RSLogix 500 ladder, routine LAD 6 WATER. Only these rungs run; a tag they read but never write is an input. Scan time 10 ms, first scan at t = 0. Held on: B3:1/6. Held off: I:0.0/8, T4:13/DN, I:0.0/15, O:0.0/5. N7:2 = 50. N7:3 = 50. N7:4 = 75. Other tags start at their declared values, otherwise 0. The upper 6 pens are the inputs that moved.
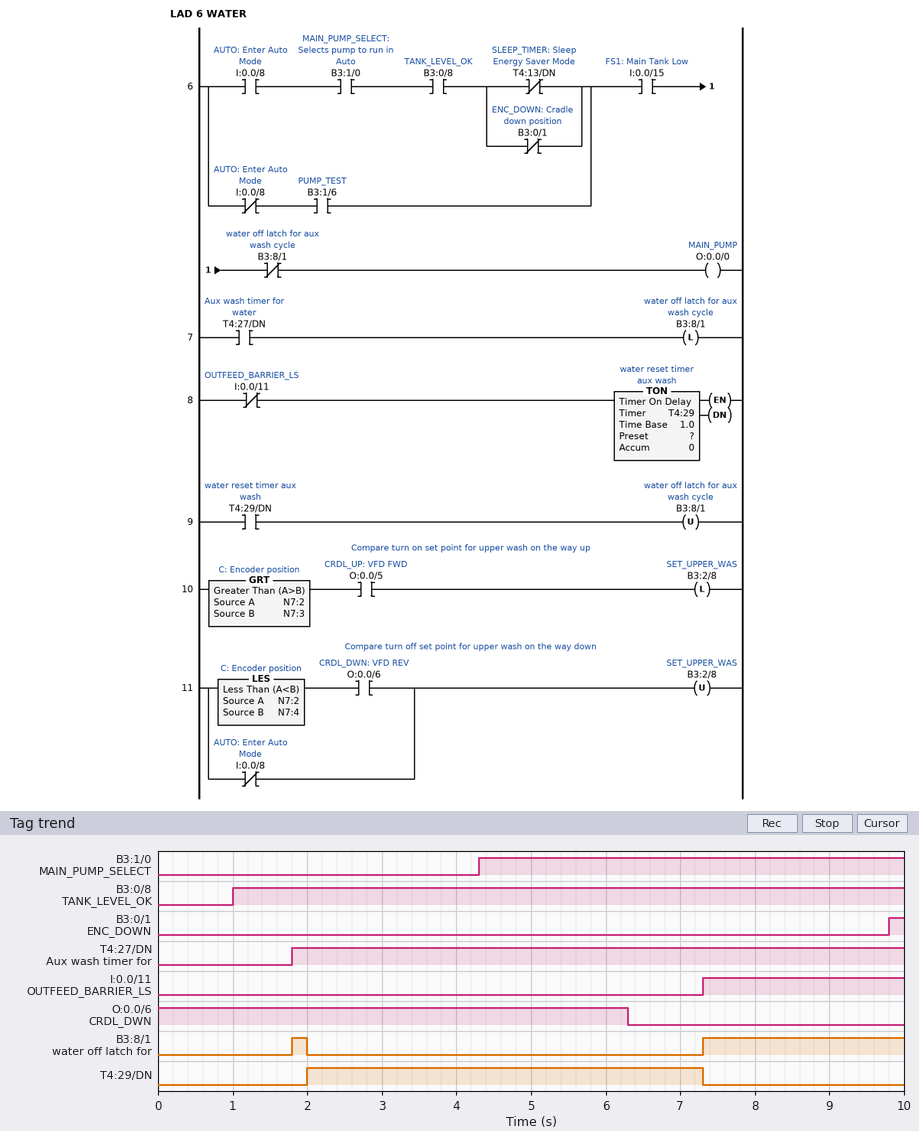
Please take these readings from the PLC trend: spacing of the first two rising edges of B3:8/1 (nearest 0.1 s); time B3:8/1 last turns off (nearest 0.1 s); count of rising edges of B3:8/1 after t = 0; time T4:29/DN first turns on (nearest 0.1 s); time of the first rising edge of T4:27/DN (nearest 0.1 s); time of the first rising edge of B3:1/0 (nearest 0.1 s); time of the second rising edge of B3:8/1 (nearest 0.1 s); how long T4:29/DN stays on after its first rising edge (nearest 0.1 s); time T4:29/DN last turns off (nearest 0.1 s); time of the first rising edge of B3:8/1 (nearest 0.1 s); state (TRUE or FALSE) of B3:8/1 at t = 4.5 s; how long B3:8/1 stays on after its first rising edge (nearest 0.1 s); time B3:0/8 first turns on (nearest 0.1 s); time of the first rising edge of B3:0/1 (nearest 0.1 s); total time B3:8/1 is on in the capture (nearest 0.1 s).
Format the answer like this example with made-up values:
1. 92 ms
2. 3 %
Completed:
1. 5.5 s
2. 2.0 s
3. 2
4. 2.0 s
5. 1.8 s
6. 4.3 s
7. 7.3 s
8. 5.3 s
9. 7.3 s
10. 1.8 s
11. FALSE
12. 0.2 s
13. 1.0 s
14. 9.8 s
15. 2.9 s
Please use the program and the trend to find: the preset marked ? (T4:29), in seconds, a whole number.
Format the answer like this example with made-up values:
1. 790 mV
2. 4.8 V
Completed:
1. 2 s
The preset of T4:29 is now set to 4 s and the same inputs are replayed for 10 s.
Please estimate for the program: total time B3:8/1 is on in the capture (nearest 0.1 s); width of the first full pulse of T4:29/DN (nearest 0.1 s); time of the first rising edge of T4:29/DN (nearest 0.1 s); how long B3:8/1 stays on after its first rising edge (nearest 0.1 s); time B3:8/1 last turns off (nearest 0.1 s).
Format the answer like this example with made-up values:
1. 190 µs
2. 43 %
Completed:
1. 4.9 s
2. 3.3 s
3. 4.0 s
4. 2.2 s
5. 4.0 s
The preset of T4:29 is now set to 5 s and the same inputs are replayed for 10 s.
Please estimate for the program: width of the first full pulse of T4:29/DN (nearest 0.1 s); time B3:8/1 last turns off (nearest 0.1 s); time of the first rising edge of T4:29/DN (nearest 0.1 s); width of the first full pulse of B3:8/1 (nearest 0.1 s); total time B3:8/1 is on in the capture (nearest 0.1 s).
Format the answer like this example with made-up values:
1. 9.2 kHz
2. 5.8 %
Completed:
1. 2.3 s
2. 5.0 s
3. 5.0 s
4. 3.2 s
5. 5.9 s
